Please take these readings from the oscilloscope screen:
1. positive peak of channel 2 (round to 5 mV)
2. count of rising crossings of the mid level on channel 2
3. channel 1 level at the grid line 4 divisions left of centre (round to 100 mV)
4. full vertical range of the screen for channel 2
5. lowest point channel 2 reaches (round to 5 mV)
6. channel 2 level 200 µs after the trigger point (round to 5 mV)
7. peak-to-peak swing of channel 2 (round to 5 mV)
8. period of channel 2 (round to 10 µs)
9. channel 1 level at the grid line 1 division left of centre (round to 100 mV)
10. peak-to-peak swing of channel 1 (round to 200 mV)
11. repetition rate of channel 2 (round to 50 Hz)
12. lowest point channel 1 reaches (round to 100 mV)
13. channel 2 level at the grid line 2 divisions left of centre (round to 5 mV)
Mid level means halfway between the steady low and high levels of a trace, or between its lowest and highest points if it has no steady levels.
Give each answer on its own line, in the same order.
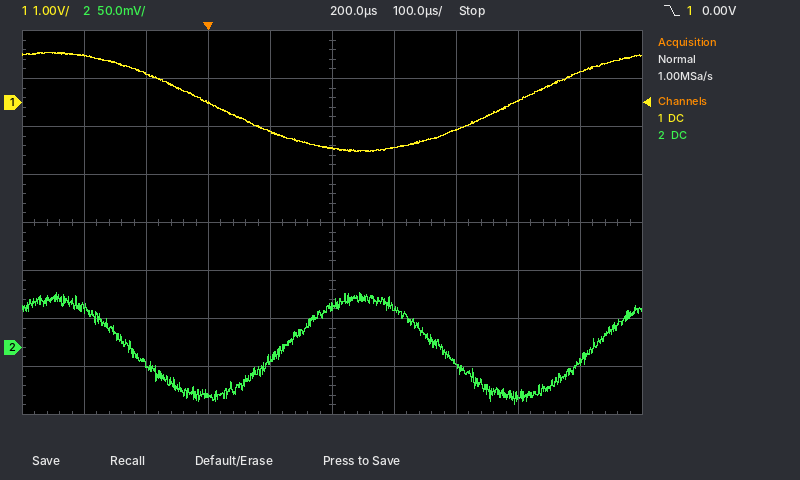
55 mV
2
1.0 V
400 mV
-60 mV
40 mV
115 mV
500 µs
-600 mV
2.0 V
2.00 kHz
-1.0 V
-50 mV
